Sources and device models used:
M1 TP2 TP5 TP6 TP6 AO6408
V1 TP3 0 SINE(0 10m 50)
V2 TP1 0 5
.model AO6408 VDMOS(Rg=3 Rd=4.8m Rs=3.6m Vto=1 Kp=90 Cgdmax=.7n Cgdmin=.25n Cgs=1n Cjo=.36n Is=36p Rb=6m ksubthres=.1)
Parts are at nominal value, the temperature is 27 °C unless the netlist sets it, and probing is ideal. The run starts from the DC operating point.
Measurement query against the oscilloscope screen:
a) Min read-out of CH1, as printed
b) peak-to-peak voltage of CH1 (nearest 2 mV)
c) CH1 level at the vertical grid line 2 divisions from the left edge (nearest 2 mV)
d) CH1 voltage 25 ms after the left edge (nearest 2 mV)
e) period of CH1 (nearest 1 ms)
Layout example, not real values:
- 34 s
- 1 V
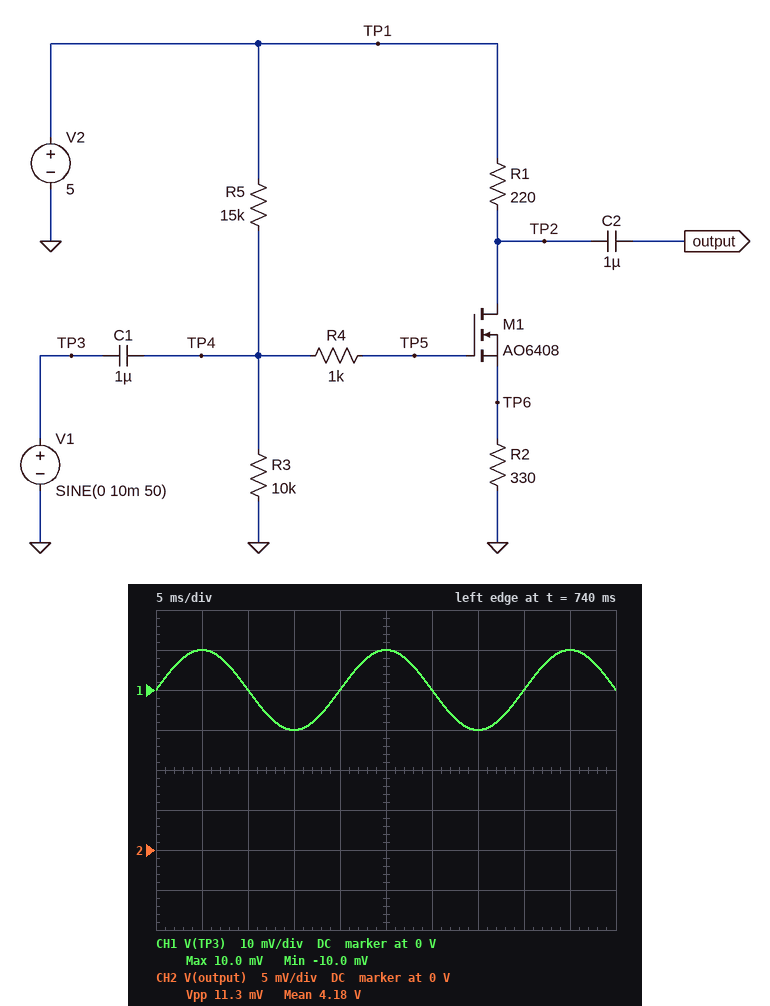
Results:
- -10.0 mV
- 20 mV
- 0 V
- 10 mV
- 20 ms
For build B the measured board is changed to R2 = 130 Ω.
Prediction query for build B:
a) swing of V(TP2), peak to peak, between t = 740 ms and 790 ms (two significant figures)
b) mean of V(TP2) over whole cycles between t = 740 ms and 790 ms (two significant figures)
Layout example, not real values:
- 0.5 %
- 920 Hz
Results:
- 29 mV
- 3.0 V
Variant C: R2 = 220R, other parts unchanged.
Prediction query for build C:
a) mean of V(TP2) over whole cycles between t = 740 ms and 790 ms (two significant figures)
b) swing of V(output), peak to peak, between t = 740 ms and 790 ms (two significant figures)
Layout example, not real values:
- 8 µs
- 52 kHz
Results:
- 3.8 V
- 17 mV
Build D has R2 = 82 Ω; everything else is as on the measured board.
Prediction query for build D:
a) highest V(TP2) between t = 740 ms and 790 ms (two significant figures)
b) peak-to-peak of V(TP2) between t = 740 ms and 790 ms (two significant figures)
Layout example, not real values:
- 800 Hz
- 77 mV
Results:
- 1.9 V
- 45 mV
